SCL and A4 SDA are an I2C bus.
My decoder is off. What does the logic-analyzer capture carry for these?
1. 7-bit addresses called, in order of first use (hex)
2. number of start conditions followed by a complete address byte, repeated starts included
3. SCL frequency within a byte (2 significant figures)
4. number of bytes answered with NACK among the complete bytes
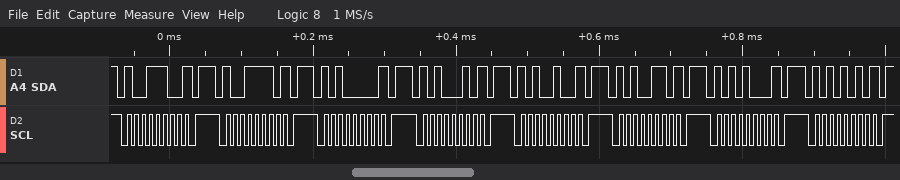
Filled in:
0x4E 0x4F 0x50 0x51 0x52 0x53 0x54 0x55
8
100 kHz
8
